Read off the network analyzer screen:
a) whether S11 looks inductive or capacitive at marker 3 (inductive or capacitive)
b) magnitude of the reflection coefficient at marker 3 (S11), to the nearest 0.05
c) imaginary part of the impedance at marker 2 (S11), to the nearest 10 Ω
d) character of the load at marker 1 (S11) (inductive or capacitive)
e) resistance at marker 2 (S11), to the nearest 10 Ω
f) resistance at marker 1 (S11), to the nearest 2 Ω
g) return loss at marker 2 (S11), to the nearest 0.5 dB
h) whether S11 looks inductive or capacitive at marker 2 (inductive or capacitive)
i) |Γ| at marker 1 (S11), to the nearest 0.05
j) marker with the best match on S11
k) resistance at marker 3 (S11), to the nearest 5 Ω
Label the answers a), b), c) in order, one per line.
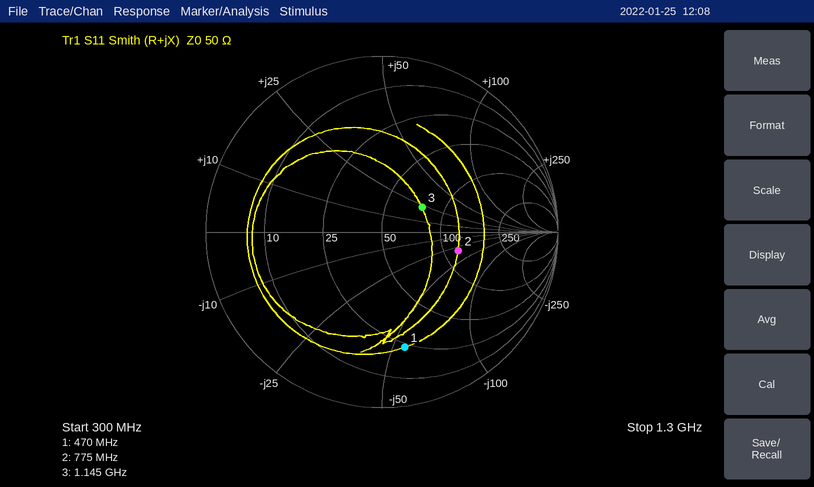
a) inductive
b) 0.25
c) -30 Ω
d) capacitive
e) 120 Ω
f) 24 Ω
g) 7.0 dB
h) capacitive
i) 0.65
j) marker 3
k) 75 Ω
